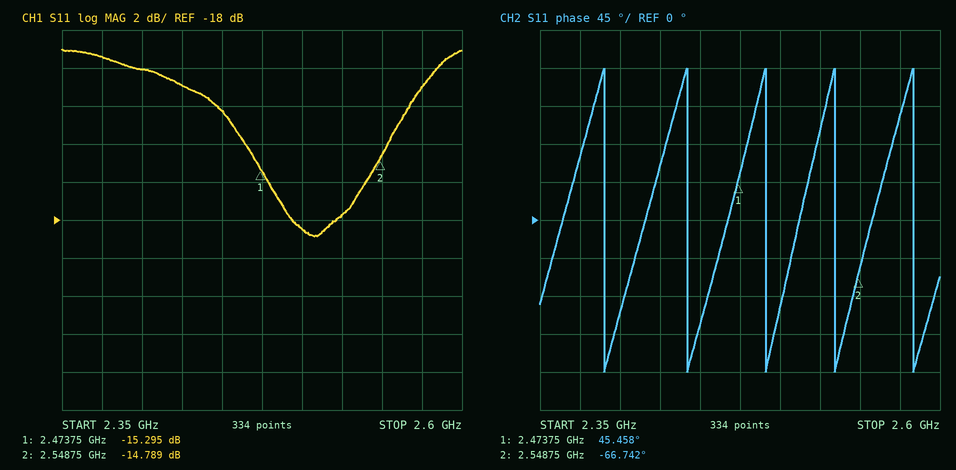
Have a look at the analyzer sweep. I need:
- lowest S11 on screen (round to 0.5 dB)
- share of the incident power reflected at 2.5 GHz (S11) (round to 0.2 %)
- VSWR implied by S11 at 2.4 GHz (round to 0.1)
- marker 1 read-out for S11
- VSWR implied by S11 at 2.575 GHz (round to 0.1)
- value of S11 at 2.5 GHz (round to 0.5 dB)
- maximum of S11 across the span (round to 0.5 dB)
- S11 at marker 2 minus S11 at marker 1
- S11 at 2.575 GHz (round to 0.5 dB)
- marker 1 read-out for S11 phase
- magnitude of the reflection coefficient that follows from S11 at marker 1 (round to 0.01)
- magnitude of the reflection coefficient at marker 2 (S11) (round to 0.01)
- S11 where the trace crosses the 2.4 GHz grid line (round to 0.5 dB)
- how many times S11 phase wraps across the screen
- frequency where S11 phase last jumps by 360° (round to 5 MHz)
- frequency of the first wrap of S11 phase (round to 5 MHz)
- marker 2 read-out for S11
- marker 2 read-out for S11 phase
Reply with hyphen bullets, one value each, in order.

- -19.0 dB
- 1.4 %
- 1.9
- -15.295 dB
- 1.8
- -18.5 dB
- -9.0 dB
- 0.506 dB
- -11.0 dB
- 45.458°
- 0.17
- 0.18
- -10.0 dB
- 5
- 2.585 GHz
- 2.390 GHz
- -14.789 dB
- -66.742°
